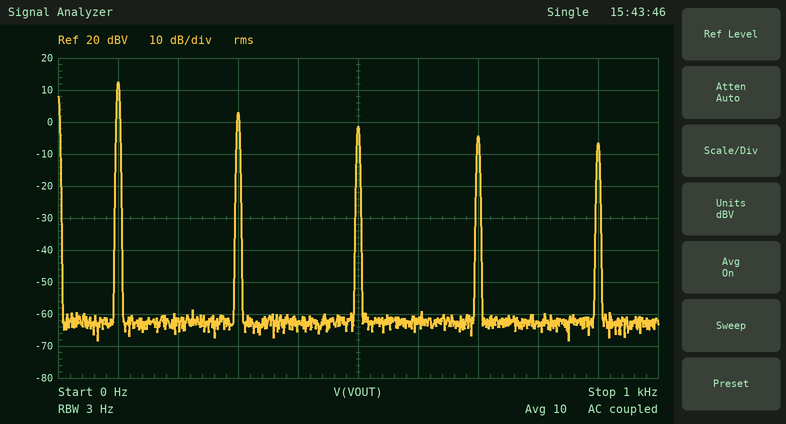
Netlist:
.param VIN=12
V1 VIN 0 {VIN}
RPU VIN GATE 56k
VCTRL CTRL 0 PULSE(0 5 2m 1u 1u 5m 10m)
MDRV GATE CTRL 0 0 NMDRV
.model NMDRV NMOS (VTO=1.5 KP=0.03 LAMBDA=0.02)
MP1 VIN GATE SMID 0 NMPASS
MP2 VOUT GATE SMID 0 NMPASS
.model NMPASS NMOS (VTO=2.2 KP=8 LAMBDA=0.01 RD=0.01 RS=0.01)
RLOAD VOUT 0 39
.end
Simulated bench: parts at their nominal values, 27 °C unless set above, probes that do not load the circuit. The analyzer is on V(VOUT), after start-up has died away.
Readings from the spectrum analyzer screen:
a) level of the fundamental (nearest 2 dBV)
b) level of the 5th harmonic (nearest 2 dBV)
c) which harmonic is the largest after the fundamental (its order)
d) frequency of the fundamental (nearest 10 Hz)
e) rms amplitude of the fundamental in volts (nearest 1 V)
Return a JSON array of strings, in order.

["12 dBV", "-2 dBV", "3", "100 Hz", "4 V"]
